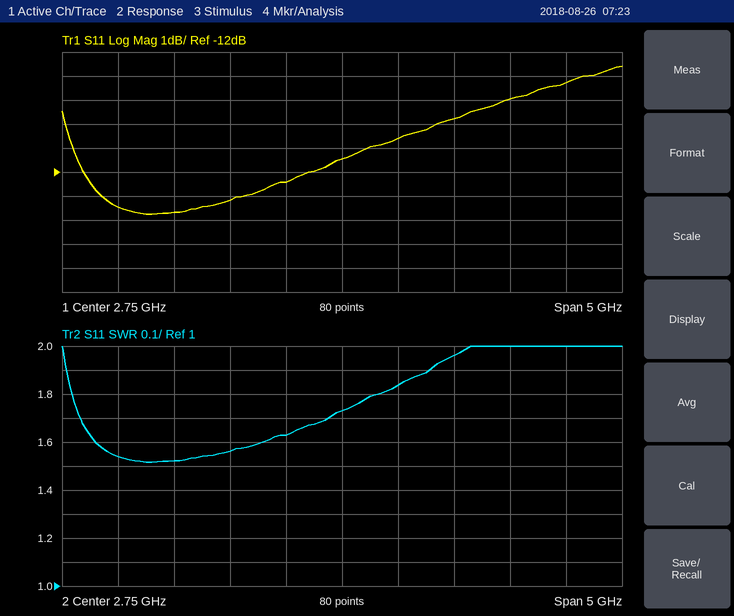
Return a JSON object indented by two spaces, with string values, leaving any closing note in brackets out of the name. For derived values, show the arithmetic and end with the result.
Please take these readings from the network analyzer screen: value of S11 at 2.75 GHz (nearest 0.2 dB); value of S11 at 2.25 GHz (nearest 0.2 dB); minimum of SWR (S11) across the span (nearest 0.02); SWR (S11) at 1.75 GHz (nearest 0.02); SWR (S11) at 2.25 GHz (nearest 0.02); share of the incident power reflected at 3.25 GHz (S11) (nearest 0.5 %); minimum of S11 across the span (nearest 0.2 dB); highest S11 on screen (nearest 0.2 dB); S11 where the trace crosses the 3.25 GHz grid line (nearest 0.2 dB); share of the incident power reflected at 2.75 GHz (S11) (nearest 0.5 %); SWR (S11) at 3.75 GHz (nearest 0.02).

{
  "value of S11 at 2.75 GHz": "-11.4 dB",
  "value of S11 at 2.25 GHz": "-12.4 dB",
  "minimum of SWR (S11) across the span": "1.52",
  "SWR (S11) at 1.75 GHz": "1.56",
  "SWR (S11) at 2.25 GHz": "1.62",
  "share of the incident power reflected at 3.25 GHz (S11)": "10^(-10.6/10) ≈ 8.71 %, so 8.5 % to the nearest 0.5 %",
  "minimum of S11 across the span": "-13.8 dB",
  "highest S11 on screen": "-7.6 dB",
  "S11 where the trace crosses the 3.25 GHz grid line": "-10.6 dB",
  "share of the incident power reflected at 2.75 GHz (S11)": "10^(-11.4/10) ≈ 7.24 %, so 7.0 % to the nearest 0.5 %",
  "SWR (S11) at 3.75 GHz": "1.96"
}
